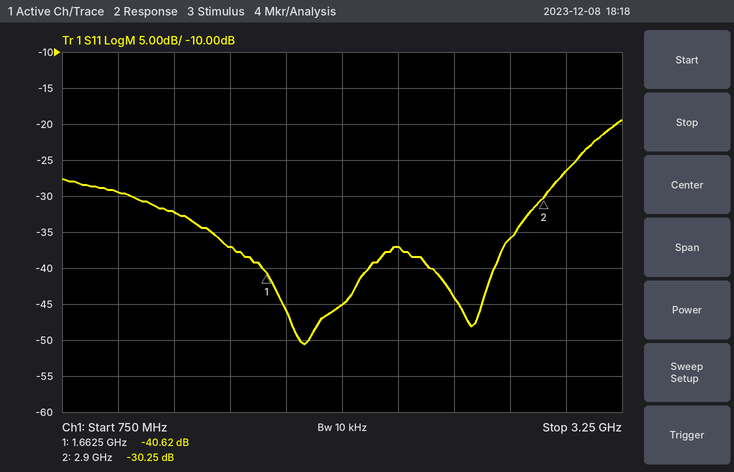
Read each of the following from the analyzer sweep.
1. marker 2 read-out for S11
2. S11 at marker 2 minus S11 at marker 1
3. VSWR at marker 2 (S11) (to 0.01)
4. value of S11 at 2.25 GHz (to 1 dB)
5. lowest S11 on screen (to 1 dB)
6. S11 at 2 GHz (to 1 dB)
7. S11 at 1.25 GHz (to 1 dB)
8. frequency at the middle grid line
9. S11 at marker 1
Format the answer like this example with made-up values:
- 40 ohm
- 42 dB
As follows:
- -30.25 dB
- 10.37 dB
- 1.06
- -37 dB
- -51 dB
- -45 dB
- -32 dB
- 2 GHz
- -40.62 dB
